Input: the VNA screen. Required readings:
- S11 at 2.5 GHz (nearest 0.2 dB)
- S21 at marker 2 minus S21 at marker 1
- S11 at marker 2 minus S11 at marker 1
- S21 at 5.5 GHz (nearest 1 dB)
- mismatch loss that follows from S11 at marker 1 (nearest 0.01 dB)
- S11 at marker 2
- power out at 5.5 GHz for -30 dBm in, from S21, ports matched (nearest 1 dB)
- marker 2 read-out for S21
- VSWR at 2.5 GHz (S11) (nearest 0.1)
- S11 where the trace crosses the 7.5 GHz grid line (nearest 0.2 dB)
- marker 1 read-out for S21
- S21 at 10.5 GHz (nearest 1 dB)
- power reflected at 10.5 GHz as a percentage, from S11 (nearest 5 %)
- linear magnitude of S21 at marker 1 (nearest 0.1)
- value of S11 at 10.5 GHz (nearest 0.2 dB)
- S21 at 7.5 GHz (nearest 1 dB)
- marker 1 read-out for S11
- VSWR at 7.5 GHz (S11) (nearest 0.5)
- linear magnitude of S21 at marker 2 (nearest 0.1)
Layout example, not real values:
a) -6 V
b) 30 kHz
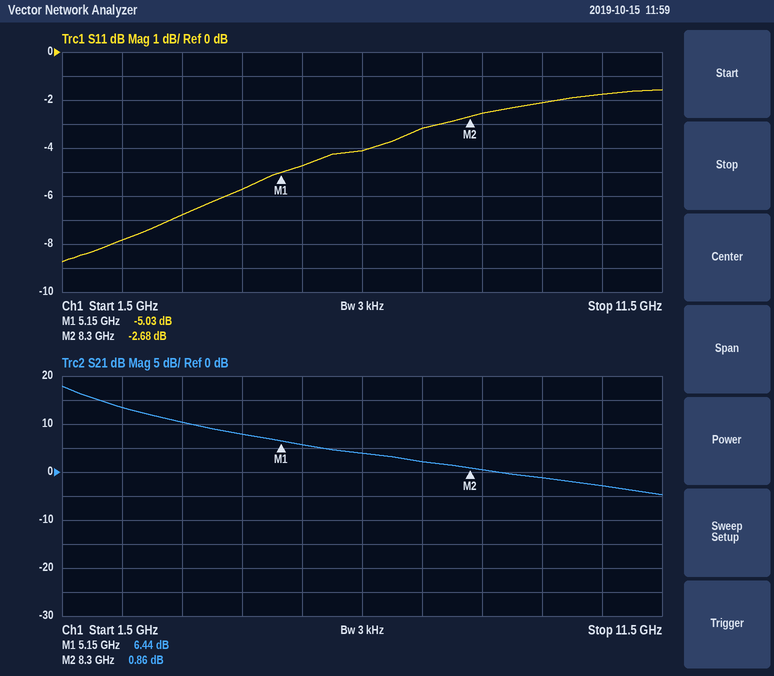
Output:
a) -7.8 dB
b) -5.58 dB
c) 2.35 dB
d) 6 dB
e) 1.64 dB
f) -2.68 dB
g) -24 dBm
h) 0.86 dB
i) 2.4
j) -3.2 dB
k) 6.44 dB
l) -3 dB
m) 65 %
n) 2.1
o) -1.8 dB
p) 2 dB
q) -5.03 dB
r) 5.5
s) 1.1
